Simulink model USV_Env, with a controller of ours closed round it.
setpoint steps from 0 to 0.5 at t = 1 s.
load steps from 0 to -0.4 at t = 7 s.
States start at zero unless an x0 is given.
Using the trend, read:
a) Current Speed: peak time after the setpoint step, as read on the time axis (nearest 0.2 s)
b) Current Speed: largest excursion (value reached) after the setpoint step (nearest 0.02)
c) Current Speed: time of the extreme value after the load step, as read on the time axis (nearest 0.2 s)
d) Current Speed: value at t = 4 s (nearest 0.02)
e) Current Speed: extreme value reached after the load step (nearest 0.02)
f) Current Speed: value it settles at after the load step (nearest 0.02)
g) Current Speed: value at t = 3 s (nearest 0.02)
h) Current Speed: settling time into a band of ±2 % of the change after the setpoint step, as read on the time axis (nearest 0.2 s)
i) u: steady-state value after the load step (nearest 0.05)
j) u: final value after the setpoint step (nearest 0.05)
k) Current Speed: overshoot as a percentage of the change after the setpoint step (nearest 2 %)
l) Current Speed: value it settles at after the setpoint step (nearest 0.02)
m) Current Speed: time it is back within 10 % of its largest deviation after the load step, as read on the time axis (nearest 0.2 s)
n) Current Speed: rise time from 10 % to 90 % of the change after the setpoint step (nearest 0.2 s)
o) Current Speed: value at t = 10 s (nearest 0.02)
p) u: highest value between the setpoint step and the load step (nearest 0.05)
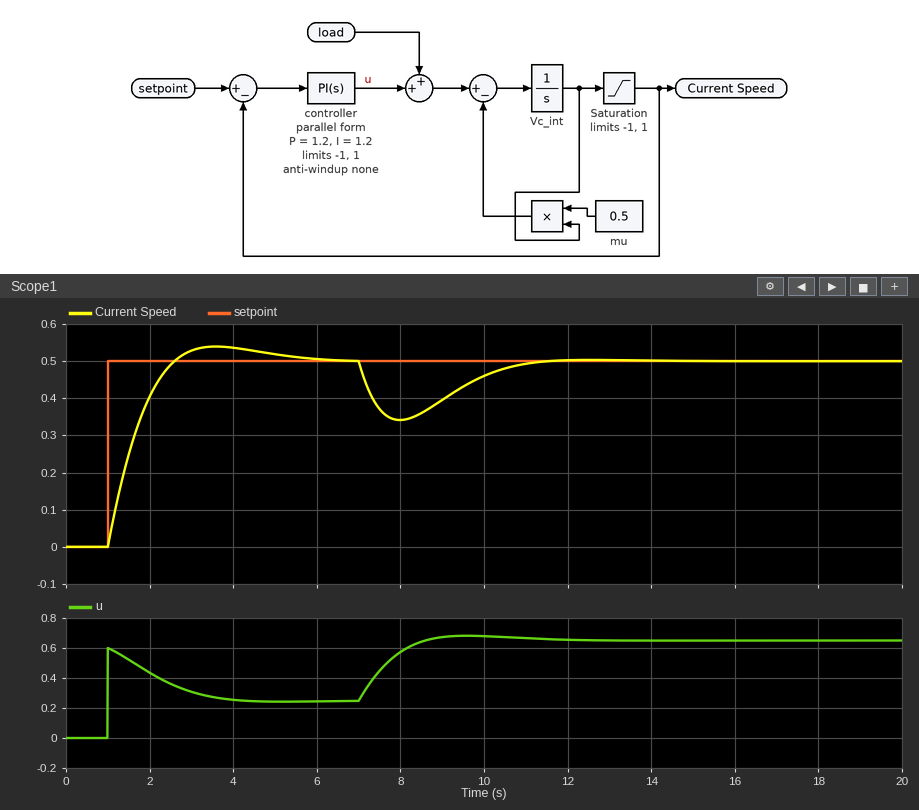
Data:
3.6 s
0.54
8.0 s
0.54
0.34
0.50
0.52
5.6 s
0.65
0.25
8 %
0.50
10.6 s
1.2 s
0.46
0.60
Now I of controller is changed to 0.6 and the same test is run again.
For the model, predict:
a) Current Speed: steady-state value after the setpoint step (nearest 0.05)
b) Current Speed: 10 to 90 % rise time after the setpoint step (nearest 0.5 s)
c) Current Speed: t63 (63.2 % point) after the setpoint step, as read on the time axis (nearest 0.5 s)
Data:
0.50
2.0 s
2.0 s
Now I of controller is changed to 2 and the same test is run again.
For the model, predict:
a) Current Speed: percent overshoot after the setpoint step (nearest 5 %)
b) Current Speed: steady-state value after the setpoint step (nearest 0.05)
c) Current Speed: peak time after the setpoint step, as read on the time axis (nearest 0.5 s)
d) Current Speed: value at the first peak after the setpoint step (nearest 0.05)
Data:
15 %
0.50
3.0 s
0.60
